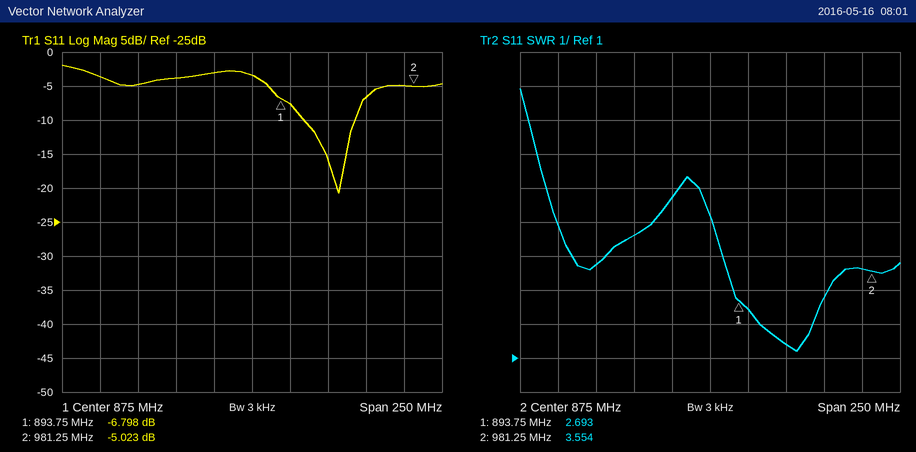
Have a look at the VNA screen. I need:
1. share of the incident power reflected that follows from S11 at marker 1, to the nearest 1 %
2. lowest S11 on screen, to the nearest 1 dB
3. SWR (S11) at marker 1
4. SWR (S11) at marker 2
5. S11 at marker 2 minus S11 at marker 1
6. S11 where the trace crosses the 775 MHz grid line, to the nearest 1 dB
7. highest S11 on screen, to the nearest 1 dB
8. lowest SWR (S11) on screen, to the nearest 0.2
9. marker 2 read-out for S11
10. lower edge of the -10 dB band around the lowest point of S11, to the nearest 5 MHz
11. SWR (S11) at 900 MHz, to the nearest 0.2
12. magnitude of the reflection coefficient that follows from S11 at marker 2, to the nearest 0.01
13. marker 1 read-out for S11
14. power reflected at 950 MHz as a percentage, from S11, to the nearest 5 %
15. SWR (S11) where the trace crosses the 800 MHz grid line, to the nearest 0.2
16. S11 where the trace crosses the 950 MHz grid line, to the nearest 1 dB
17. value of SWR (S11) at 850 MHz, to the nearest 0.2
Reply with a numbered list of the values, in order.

1. 21 %
2. -21 dB
3. 2.693
4. 3.554
5. 1.775 dB
6. -4 dB
7. -2 dB
8. 1.2
9. -5.023 dB
10. 910 MHz
11. 2.4
12. 0.56
13. -6.798 dB
14. 20 %
15. 3.8
16. -7 dB
17. 5.8
